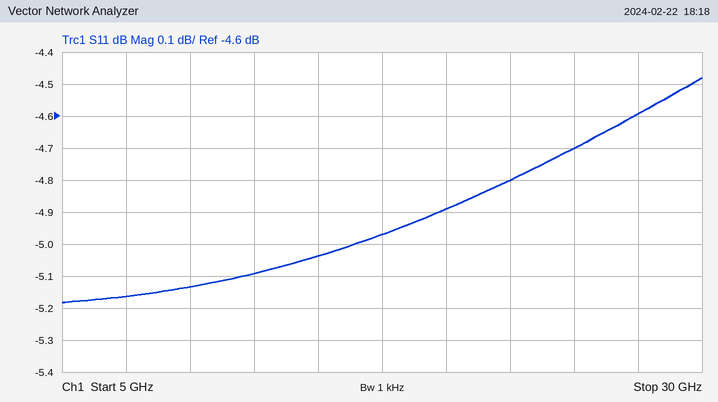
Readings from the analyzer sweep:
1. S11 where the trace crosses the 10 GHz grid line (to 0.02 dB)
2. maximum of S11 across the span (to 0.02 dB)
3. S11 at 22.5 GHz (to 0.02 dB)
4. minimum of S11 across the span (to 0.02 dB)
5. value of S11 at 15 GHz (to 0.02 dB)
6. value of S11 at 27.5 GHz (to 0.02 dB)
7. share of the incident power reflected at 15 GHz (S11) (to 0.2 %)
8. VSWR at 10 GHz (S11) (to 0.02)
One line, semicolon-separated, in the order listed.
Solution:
-5.14 dB; -4.48 dB; -4.80 dB; -5.18 dB; -5.04 dB; -4.60 dB; 31.4 %; 3.48
